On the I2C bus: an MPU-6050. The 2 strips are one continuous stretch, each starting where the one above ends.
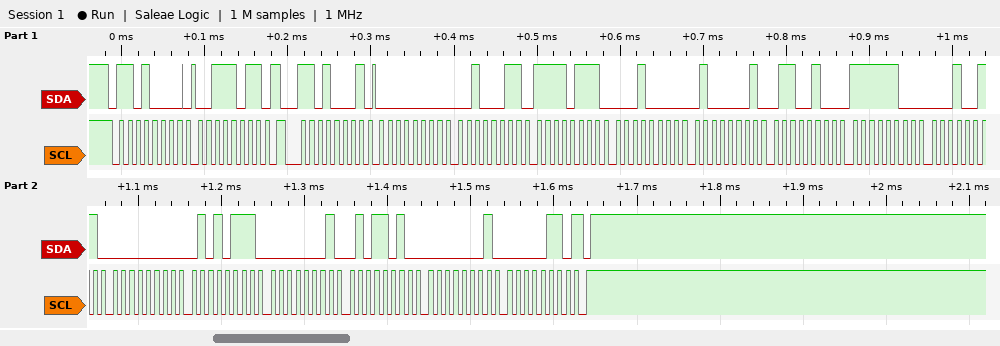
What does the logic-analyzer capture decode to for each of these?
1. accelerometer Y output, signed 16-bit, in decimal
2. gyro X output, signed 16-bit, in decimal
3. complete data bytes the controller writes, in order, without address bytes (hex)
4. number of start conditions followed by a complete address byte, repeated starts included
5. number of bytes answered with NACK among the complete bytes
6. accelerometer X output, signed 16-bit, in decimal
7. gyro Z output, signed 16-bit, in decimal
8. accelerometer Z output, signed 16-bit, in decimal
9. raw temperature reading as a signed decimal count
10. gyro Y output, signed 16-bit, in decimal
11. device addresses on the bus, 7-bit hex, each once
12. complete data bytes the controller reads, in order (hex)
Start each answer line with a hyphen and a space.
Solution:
- -2288
- 87
- 3B
- 2
- 1
- 35
- 262
- 16740
- -1005
- 346
- 0x68
- 00 23 F7 10 41 64 FC 13 00 57 01 5A 01 06
